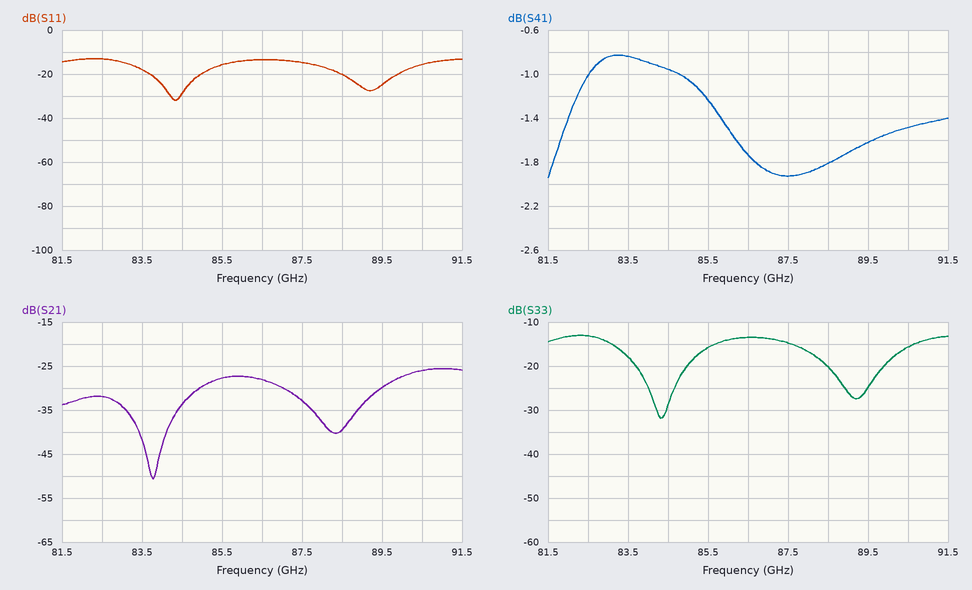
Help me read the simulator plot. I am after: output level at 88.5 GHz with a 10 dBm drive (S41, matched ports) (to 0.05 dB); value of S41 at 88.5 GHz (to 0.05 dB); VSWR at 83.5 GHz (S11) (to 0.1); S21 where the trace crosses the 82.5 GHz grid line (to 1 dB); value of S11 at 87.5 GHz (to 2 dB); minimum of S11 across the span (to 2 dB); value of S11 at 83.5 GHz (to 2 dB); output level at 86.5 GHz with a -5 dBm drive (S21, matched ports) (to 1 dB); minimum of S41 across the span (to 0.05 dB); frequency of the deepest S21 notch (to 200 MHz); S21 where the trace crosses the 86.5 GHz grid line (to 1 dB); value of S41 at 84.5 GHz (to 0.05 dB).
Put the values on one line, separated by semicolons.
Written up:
8.20 dBm; -1.80 dB; 1.3; -32 dB; -14 dB; -32 dB; -18 dB; -33 dBm; -1.95 dB; 83.8 GHz; -28 dB; -0.95 dB
